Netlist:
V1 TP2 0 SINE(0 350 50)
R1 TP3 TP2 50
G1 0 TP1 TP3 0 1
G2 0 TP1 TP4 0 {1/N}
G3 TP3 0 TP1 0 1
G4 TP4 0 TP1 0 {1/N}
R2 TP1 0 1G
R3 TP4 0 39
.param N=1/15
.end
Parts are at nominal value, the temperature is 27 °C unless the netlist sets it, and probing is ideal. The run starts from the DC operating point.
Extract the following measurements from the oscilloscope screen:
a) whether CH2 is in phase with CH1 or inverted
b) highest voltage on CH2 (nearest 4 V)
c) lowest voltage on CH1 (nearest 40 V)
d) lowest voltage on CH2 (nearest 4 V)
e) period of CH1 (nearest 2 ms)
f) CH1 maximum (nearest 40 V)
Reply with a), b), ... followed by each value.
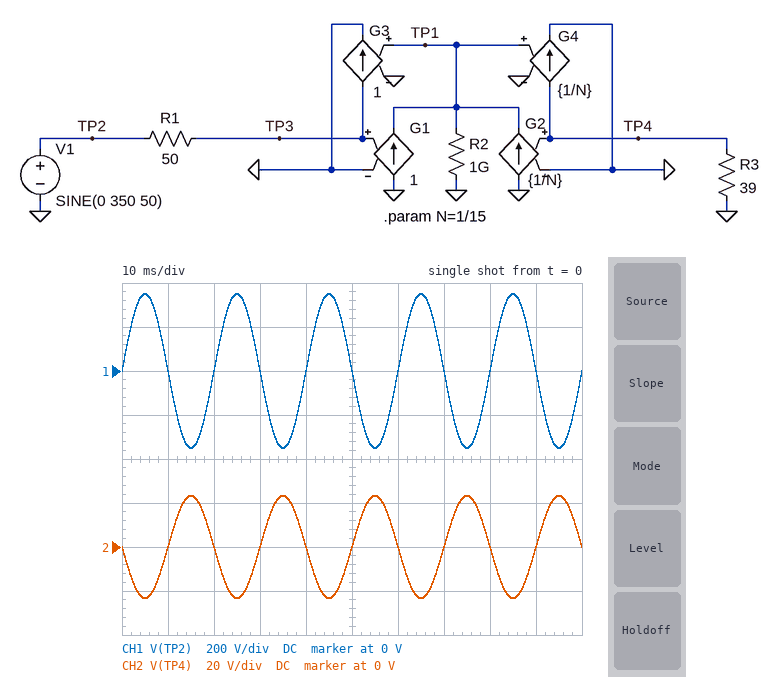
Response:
a) inverted
b) 24 V
c) -360 V
d) -24 V
e) 20 ms
f) 360 V
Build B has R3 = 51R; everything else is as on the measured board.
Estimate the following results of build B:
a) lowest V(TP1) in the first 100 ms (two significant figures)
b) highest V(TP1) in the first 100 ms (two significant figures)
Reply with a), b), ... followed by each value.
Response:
a) -30 mV
b) 30 mV
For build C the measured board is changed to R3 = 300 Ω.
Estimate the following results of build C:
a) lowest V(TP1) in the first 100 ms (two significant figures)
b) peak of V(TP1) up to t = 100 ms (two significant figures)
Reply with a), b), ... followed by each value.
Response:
a) -5.2 mV
b) 5.2 mV
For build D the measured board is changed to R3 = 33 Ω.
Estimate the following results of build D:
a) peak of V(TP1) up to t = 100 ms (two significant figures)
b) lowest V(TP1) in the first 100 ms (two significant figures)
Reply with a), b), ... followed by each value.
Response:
a) 47 mV
b) -47 mV
